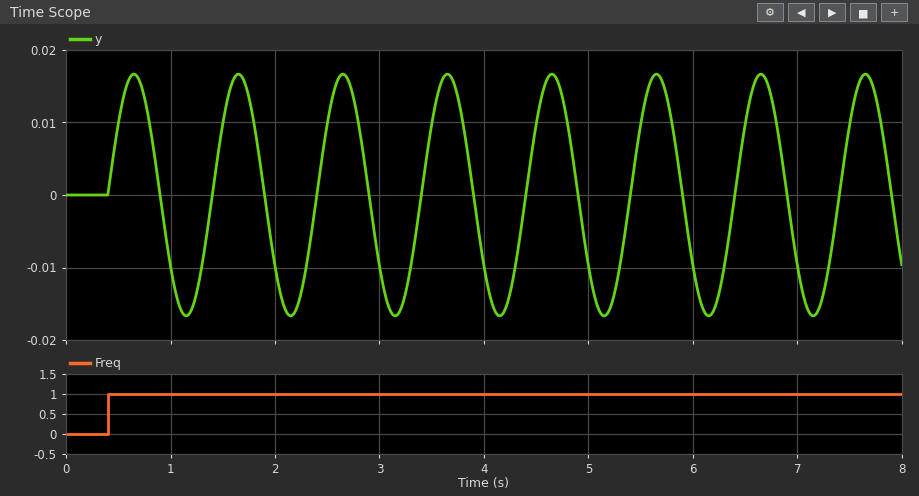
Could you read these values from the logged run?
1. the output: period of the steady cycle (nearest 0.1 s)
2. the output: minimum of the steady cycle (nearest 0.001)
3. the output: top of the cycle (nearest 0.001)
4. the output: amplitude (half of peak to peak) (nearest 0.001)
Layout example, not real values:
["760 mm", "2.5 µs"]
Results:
["1.0 s", "-0.017", "0.017", "0.017"]
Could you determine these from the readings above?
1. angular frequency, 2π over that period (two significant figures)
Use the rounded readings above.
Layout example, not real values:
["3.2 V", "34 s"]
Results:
["6.3 rad/s"]
